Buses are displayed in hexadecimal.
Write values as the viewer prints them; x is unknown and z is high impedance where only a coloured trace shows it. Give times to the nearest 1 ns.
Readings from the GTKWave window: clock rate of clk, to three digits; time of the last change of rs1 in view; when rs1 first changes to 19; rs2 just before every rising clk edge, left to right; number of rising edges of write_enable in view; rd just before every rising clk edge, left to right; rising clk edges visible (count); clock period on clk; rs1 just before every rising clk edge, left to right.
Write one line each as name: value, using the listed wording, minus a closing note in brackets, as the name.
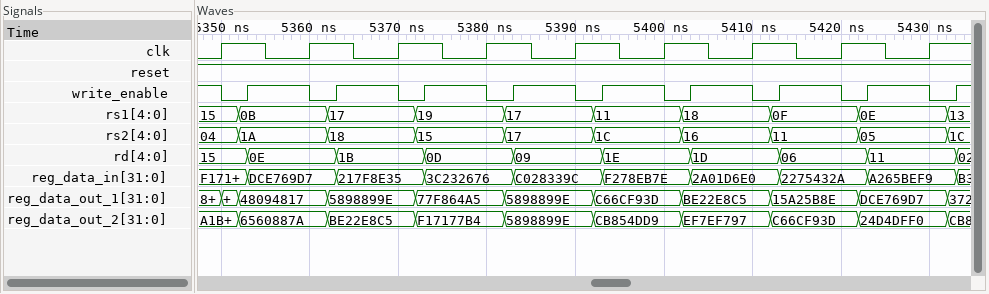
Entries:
clock rate of clk, to three digits: 100 MHz
time of the last change of rs1 in view: 5432 ns
when rs1 first changes to 19: 5372 ns
rs2 just before every rising clk edge, left to right: 04, 1A, 18, 15, 17, 1C, 16, 11, 05
number of rising edges of write_enable in view: 9
rd just before every rising clk edge, left to right: 15, 0E, 1B, 0D, 09, 1E, 1D, 06, 11
rising clk edges visible: 9
clock period on clk: 10 ns
rs1 just before every rising clk edge, left to right: 15, 0B, 17, 19, 17, 11, 18, 0F, 0E
